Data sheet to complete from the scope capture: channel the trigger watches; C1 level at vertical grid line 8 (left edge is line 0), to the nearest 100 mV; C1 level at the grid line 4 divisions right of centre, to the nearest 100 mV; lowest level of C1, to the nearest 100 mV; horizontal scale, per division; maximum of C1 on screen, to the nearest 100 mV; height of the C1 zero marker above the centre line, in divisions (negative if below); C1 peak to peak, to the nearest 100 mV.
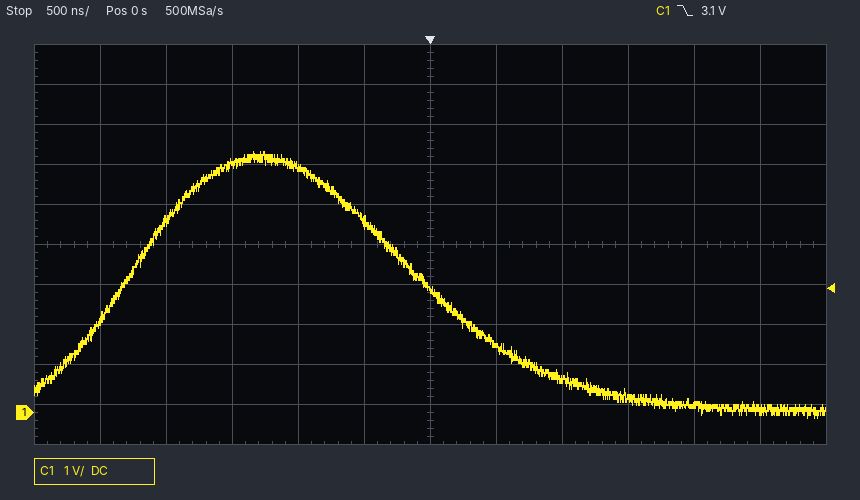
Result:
C1
800 mV
200 mV
-100 mV
500 ns
6.5 V
-4.2 div
6.6 V
